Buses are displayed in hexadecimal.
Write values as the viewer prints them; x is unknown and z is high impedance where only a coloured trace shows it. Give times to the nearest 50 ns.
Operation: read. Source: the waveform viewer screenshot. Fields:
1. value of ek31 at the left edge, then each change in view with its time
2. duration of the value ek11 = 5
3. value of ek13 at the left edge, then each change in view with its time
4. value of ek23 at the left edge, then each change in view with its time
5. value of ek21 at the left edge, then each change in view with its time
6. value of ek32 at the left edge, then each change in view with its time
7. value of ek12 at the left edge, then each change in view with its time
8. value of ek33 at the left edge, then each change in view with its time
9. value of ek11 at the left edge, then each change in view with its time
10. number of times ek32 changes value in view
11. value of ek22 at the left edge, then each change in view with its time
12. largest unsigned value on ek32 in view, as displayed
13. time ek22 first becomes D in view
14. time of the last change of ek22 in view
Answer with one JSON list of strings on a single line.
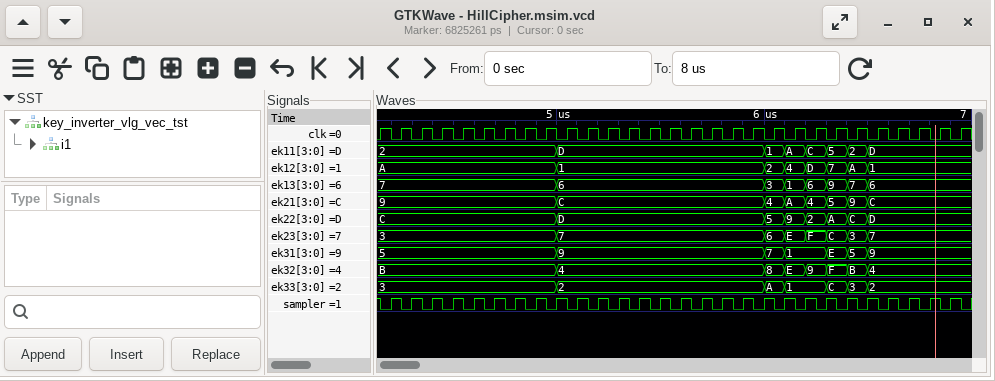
["5, 9 at 5000 ns, 7 at 6000 ns, 1 at 6100 ns, E at 6300 ns, 5 at 6400 ns, 9 at 6500 ns", "100 ns", "7, 6 at 5000 ns, 3 at 6000 ns, 1 at 6100 ns, 6 at 6200 ns, 9 at 6300 ns, 7 at 6400 ns, 6 at 6500 ns", "3, 7 at 5000 ns, 6 at 6000 ns, E at 6100 ns, F at 6200 ns, C at 6300 ns, 3 at 6400 ns, 7 at 6500 ns", "9, C at 5000 ns, 4 at 6000 ns, A at 6100 ns, 4 at 6200 ns, 5 at 6300 ns, 9 at 6400 ns, C at 6500 ns", "B, 4 at 5000 ns, 8 at 6000 ns, E at 6100 ns, 9 at 6200 ns, F at 6300 ns, B at 6400 ns, 4 at 6500 ns", "A, 1 at 5000 ns, 2 at 6000 ns, 4 at 6100 ns, D at 6200 ns, 7 at 6300 ns, A at 6400 ns, 1 at 6500 ns", "3, 2 at 5000 ns, A at 6000 ns, 1 at 6100 ns, C at 6300 ns, 3 at 6400 ns, 2 at 6500 ns", "2, D at 5000 ns, 1 at 6000 ns, A at 6100 ns, C at 6200 ns, 5 at 6300 ns, 2 at 6400 ns, D at 6500 ns", "7", "C, D at 5000 ns, 5 at 6000 ns, 9 at 6100 ns, 2 at 6200 ns, A at 6300 ns, C at 6400 ns, D at 6500 ns", "F", "5000 ns", "6500 ns"]
